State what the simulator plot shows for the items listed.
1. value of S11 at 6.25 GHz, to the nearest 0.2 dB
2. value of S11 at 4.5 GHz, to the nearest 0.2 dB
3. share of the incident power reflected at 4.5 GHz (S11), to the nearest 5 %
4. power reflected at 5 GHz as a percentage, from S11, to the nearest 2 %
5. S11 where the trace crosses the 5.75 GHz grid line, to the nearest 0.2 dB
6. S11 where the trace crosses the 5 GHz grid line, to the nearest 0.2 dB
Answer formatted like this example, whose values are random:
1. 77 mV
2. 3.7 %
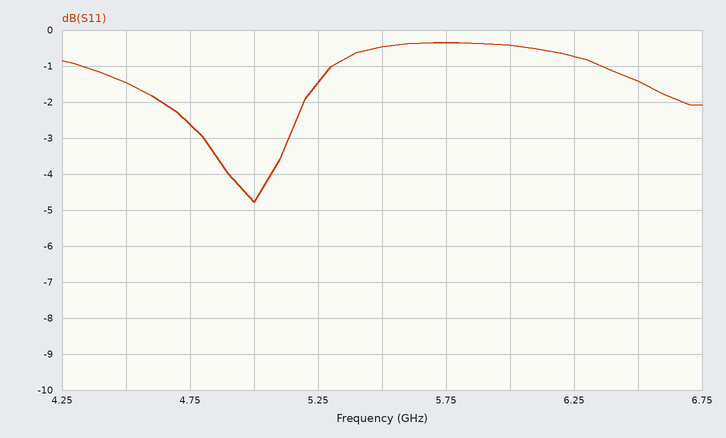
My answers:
1. -0.8 dB
2. -1.4 dB
3. 70 %
4. 34 %
5. -0.4 dB
6. -4.8 dB
